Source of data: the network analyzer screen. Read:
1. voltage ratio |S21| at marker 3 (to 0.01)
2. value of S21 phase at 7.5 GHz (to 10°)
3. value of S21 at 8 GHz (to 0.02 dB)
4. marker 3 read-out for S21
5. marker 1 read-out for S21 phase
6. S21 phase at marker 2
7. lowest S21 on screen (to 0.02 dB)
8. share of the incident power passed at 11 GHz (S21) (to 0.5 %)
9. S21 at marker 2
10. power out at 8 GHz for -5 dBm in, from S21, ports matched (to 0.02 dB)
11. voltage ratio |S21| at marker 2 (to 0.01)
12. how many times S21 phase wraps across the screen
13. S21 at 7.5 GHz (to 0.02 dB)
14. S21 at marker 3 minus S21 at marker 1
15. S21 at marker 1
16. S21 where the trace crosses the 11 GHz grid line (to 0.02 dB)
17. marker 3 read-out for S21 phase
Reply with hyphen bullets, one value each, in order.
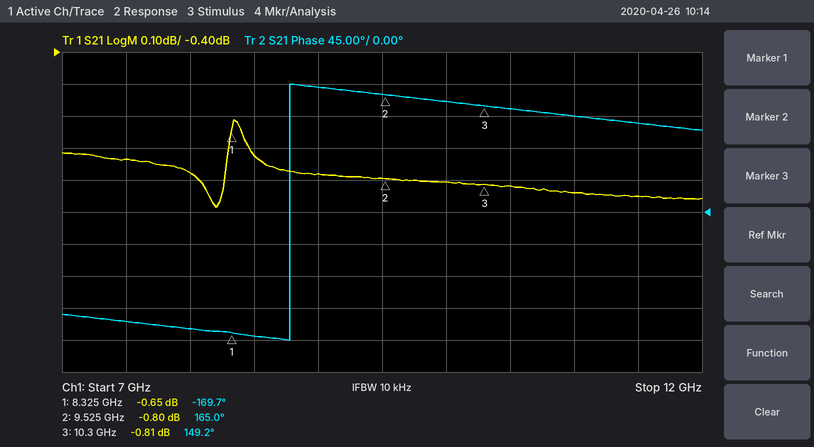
- 0.91
- -150°
- -0.78 dB
- -0.81 dB
- -169.7°
- 165.0°
- -0.88 dB
- 82.5 %
- -0.80 dB
- -5.78 dBm
- 0.91
- 1
- -0.74 dB
- -0.16 dB
- -0.65 dB
- -0.84 dB
- 149.2°
